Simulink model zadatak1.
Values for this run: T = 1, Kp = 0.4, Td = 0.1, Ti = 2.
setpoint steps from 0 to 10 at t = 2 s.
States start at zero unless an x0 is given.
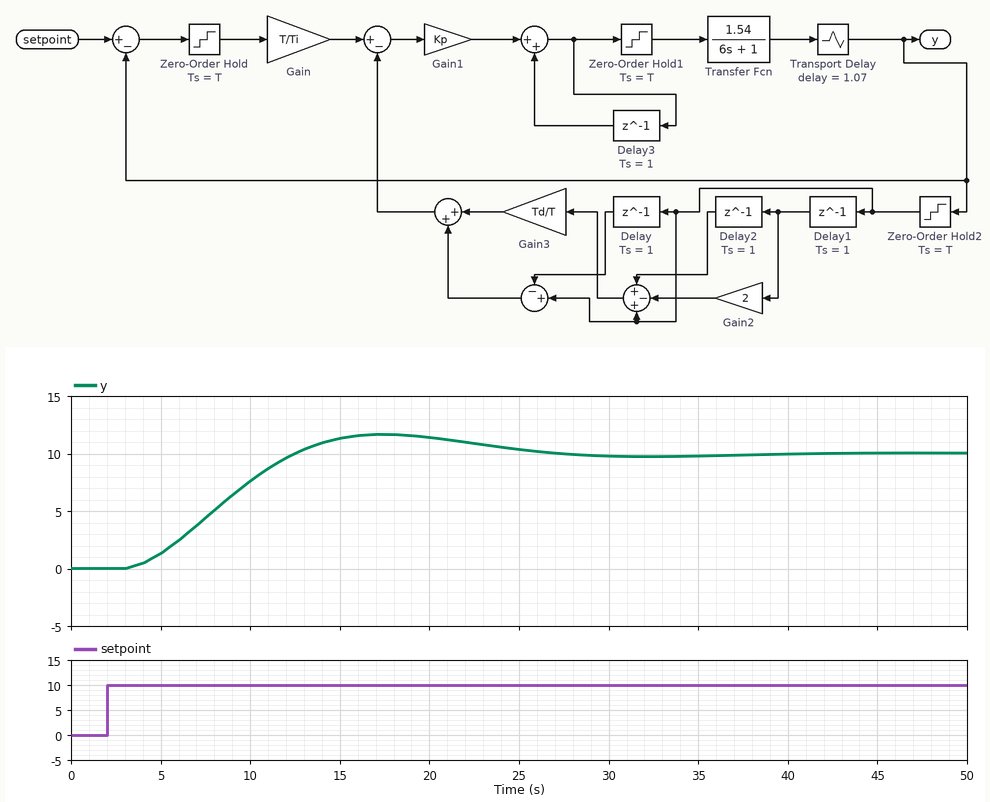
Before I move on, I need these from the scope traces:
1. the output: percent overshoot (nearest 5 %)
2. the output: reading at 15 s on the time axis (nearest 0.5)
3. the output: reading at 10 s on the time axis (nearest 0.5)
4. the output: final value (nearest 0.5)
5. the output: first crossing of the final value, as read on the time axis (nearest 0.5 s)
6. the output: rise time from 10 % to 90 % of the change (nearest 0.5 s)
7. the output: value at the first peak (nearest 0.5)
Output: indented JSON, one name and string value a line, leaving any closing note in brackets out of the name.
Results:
{
  "the output: percent overshoot": "15 %",
  "the output: reading at 15 s on the time axis": "11.5",
  "the output: reading at 10 s on the time axis": "7.5",
  "the output: final value": "10.0",
  "the output: first crossing of the final value, as read on the time axis": "12.5 s",
  "the output: rise time from 10 % to 90 % of the change": "6.5 s",
  "the output: value at the first peak": "11.5"
}
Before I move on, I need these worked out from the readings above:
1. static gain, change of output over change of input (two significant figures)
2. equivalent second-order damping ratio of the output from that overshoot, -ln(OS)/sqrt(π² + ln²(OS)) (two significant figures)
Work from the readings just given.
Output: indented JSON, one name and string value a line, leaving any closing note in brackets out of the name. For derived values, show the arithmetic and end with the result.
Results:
{
  "static gain, change of output over change of input": "(10 - 0) / (10 - 0) = 1.0",
  "equivalent second-order damping ratio of the output from that overshoot, -ln(OS)/sqrt(π² + ln²(OS))": "ln(0.15) = -1.897; 1.897 / sqrt(9.870 + 3.599) = 0.52"
}
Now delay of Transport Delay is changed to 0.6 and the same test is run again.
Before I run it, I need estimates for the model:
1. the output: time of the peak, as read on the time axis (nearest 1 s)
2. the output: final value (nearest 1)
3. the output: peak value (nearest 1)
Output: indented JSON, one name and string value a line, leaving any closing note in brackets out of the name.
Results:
{
  "the output: time of the peak, as read on the time axis": "18 s",
  "the output: final value": "10",
  "the output: peak value": "11"
}
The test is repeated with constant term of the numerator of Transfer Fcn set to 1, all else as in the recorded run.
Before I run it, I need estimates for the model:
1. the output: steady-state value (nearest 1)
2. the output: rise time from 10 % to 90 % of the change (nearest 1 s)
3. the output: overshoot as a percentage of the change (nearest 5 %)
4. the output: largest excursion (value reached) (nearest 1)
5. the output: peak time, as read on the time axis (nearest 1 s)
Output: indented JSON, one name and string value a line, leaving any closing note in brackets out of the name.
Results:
{
  "the output: steady-state value": "10",
  "the output: rise time from 10 % to 90 % of the change": "9 s",
  "the output: overshoot as a percentage of the change": "10 %",
  "the output: largest excursion (value reached)": "11",
  "the output: peak time, as read on the time axis": "22 s"
}
